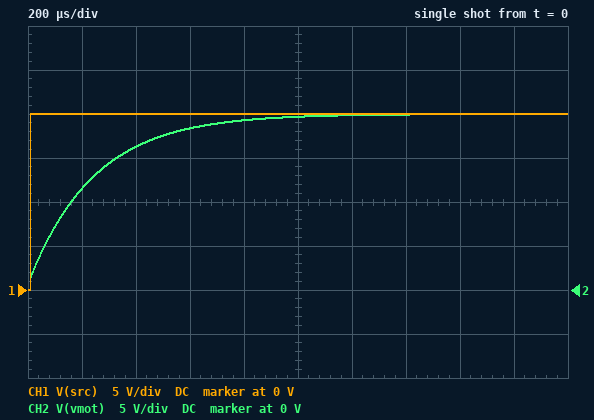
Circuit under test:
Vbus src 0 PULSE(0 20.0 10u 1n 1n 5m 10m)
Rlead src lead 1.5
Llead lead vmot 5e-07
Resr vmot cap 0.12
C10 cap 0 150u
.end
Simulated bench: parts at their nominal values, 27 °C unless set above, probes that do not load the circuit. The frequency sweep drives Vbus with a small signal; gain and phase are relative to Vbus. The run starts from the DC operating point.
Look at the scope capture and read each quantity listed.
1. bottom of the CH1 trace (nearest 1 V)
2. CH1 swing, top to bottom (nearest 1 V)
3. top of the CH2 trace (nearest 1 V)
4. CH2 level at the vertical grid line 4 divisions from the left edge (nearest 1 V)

0 V
20 V
20 V
19 V
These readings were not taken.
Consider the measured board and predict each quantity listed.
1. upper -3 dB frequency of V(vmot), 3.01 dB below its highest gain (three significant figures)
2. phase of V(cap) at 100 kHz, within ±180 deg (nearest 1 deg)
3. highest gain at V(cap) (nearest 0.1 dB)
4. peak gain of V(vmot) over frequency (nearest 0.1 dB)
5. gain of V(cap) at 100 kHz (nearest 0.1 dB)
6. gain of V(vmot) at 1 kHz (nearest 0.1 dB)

659 Hz
-101 deg
0 dB
0 dB
-43.8 dB
-5.2 dB
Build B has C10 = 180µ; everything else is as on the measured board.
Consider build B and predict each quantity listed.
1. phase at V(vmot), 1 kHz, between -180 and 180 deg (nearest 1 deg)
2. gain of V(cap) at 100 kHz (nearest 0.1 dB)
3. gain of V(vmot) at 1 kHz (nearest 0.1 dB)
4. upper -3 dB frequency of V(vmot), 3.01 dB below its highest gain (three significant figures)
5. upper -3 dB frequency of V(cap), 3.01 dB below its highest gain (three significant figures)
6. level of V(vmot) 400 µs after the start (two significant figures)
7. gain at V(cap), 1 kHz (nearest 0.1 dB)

-54 deg
-45.4 dB
-6.3 dB
549 Hz
546 Hz
15 V
-6.4 dB
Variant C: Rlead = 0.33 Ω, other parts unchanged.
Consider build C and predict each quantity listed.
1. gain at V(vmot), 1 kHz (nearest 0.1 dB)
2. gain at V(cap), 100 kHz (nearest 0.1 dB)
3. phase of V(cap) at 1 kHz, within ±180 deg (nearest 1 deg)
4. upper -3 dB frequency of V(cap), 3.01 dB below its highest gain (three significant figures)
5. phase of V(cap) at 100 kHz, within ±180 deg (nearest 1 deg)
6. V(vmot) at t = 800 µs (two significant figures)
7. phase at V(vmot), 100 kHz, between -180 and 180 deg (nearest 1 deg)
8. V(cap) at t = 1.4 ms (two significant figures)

-0.6 dB
-34.2 dB
-23 deg
2.40 kHz
-124 deg
20 V
-39 deg
20 V
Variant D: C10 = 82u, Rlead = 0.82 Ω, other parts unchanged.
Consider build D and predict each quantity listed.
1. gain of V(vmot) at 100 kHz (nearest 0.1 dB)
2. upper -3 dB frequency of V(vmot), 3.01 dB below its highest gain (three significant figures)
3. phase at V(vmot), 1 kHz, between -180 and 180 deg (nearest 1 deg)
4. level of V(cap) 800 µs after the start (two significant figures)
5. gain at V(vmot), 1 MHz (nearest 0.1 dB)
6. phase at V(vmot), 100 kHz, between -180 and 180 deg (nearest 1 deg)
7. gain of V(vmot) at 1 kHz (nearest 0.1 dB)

-18.2 dB
2.11 kHz
-22 deg
20 V
-28.7 dB
-27 deg
-0.9 dB
